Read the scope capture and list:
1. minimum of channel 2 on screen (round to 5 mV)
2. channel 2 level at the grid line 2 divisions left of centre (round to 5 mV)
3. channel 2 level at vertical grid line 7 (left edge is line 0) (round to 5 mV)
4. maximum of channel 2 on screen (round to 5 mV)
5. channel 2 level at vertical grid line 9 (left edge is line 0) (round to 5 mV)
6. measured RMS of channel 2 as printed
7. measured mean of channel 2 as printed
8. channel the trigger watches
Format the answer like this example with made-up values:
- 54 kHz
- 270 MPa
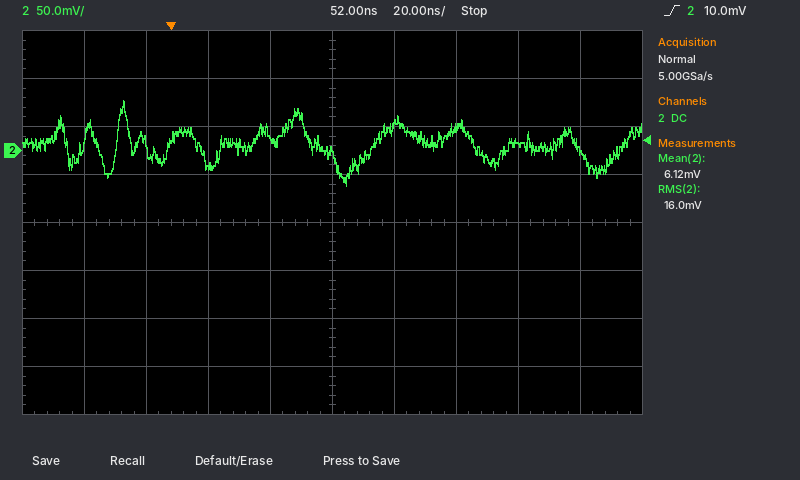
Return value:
- -35 mV
- -15 mV
- 25 mV
- 50 mV
- 0 mV
- 16.0 mV
- 6.12 mV
- channel 2
